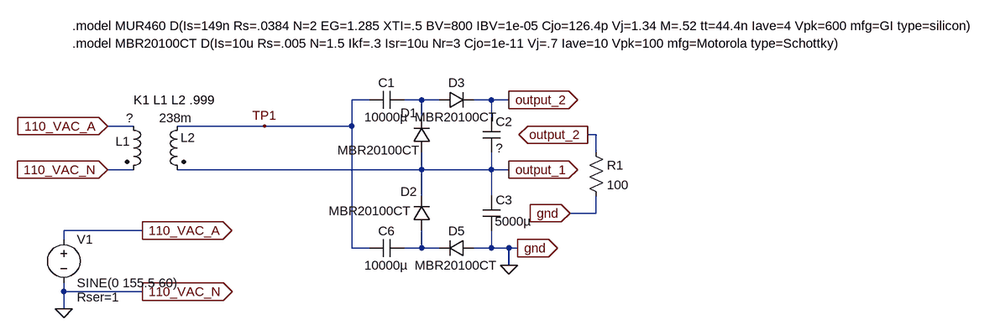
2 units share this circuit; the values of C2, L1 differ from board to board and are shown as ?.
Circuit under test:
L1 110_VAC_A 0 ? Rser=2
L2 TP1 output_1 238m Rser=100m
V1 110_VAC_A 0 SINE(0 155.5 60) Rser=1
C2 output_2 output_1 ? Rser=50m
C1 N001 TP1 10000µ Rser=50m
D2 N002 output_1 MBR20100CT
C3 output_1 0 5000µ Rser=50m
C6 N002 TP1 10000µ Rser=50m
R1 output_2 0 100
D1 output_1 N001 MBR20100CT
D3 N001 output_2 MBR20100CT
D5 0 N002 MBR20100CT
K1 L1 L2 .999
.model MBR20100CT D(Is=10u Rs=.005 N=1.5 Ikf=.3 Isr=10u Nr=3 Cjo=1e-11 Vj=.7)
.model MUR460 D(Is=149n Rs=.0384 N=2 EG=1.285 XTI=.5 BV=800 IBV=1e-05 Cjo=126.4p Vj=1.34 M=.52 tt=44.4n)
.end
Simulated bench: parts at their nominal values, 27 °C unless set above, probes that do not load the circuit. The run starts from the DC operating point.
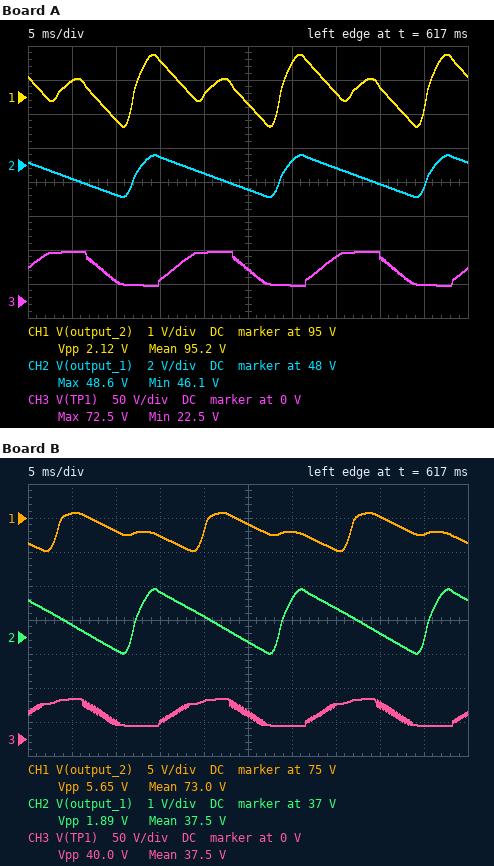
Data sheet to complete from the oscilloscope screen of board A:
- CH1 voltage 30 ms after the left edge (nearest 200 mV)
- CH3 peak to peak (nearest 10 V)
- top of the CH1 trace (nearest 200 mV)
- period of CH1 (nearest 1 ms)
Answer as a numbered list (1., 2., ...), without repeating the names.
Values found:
1. 96.0 V
2. 50 V
3. 96.2 V
4. 17 ms
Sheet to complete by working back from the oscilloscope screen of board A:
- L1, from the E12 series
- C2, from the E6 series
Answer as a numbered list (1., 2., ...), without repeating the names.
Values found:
1. 6.8 H
2. 10 mF
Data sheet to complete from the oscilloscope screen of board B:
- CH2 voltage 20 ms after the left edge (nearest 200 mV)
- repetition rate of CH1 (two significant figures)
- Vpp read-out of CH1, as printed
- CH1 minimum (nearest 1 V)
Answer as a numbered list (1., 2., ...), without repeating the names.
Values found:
1. 37.6 V
2. 60 Hz
3. 5.65 V
4. 70 V
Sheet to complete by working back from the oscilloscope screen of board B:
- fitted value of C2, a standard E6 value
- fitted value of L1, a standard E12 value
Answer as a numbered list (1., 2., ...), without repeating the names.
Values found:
1. 1.5 mF
2. 12 H
